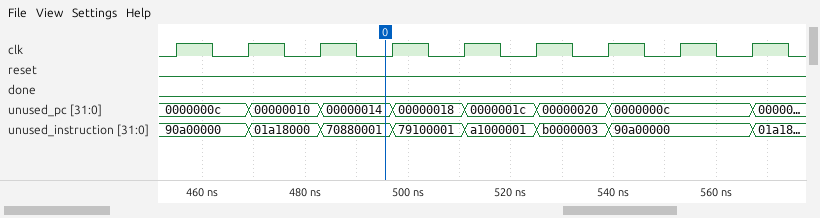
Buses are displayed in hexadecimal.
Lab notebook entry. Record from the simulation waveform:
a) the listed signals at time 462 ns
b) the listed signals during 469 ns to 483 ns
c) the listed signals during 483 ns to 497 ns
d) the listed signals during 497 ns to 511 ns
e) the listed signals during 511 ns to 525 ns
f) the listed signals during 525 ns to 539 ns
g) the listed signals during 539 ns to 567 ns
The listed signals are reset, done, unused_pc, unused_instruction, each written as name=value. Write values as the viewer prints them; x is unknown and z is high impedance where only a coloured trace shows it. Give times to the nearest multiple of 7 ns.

reset=0, done=0, unused_pc=0000000c, unused_instruction=90a00000
reset=0, done=0, unused_pc=00000010, unused_instruction=01a18000
reset=0, done=0, unused_pc=00000014, unused_instruction=70880001
reset=0, done=0, unused_pc=00000018, unused_instruction=79100001
reset=0, done=0, unused_pc=0000001c, unused_instruction=a1000001
reset=0, done=0, unused_pc=00000020, unused_instruction=b0000003
reset=0, done=0, unused_pc=0000000c, unused_instruction=90a00000
